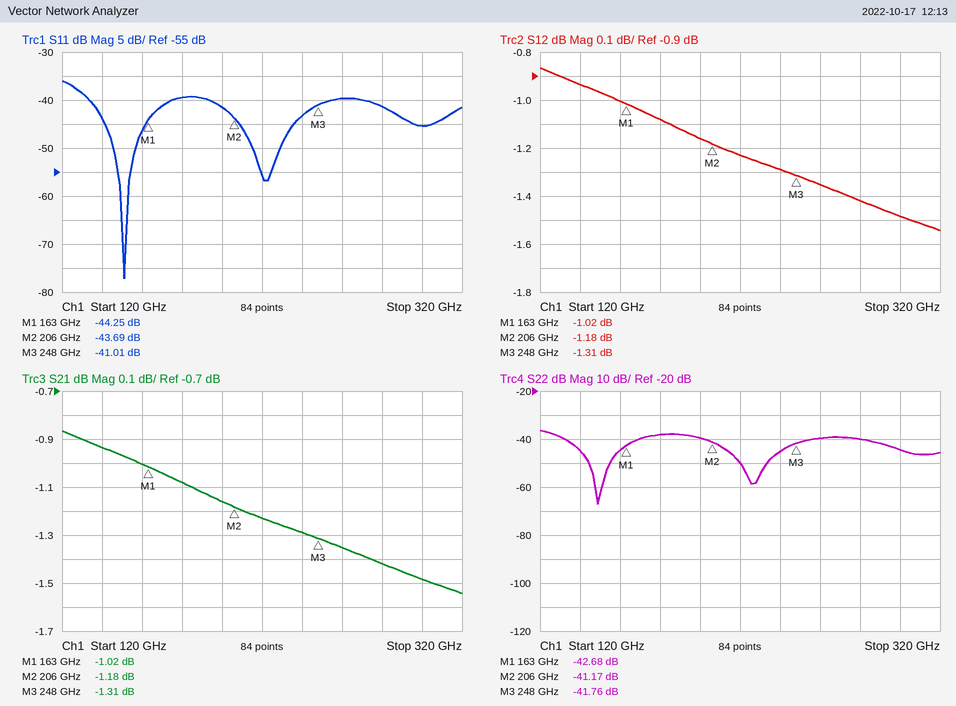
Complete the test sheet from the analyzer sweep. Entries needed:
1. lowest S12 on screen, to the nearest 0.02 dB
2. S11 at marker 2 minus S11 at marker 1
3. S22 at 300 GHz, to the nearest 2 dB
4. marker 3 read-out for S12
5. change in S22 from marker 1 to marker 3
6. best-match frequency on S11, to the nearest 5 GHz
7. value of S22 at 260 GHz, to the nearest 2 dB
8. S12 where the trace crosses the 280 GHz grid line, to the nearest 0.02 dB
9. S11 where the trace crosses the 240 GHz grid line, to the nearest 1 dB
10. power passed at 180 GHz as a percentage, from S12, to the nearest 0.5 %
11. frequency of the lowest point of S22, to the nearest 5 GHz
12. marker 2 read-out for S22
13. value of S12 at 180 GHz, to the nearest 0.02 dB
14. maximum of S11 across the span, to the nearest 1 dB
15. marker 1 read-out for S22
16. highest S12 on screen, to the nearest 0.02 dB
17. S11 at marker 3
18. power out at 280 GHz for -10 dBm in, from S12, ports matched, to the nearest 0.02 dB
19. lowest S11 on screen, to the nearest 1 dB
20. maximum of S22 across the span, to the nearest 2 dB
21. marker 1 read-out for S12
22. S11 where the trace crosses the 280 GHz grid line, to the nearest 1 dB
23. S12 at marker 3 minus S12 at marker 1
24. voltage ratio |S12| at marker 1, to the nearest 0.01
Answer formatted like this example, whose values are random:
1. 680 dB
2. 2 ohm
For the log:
1. -1.54 dB
2. 0.56 dB
3. -44 dB
4. -1.31 dB
5. 0.92 dB
6. 150 GHz
7. -40 dB
8. -1.42 dB
9. -43 dB
10. 78.0 %
11. 150 GHz
12. -41.17 dB
13. -1.08 dB
14. -36 dB
15. -42.68 dB
16. -0.86 dB
17. -41.01 dB
18. -11.42 dBm
19. -77 dB
20. -36 dB
21. -1.02 dB
22. -41 dB
23. -0.29 dB
24. 0.89
